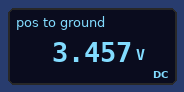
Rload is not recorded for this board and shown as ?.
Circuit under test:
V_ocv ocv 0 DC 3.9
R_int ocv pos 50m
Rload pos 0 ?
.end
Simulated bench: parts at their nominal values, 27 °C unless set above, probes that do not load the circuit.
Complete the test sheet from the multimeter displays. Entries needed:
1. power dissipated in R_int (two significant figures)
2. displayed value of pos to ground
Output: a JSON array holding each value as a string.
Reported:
["3.9 W", "3.457 V"]
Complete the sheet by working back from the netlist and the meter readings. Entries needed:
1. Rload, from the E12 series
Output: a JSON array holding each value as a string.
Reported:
["0.39 Ω"]
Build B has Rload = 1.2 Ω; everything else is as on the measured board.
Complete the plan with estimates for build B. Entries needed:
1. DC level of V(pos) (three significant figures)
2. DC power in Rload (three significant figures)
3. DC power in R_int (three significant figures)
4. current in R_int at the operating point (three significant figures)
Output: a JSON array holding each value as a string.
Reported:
["3.74 V", "11.7 W", "487 mW", "3.12 A"]
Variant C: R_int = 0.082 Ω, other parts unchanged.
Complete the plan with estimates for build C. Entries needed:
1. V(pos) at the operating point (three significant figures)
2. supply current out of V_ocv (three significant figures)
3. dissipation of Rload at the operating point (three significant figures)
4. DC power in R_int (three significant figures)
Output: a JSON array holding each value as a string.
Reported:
["3.22 V", "8.26 A", "26.6 W", "5.60 W"]
